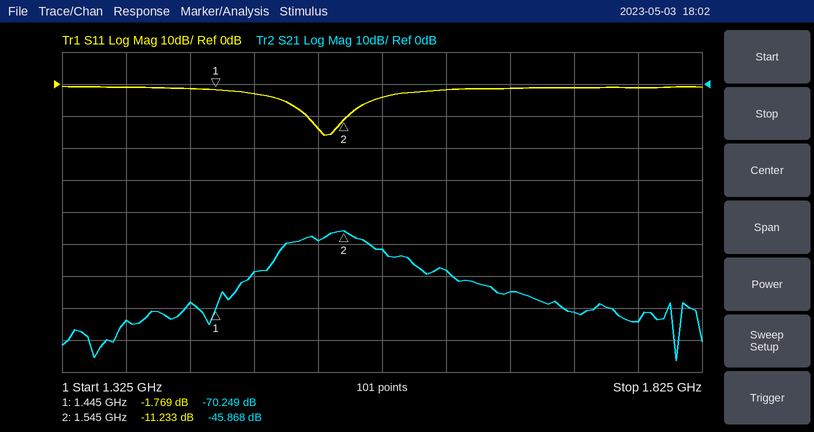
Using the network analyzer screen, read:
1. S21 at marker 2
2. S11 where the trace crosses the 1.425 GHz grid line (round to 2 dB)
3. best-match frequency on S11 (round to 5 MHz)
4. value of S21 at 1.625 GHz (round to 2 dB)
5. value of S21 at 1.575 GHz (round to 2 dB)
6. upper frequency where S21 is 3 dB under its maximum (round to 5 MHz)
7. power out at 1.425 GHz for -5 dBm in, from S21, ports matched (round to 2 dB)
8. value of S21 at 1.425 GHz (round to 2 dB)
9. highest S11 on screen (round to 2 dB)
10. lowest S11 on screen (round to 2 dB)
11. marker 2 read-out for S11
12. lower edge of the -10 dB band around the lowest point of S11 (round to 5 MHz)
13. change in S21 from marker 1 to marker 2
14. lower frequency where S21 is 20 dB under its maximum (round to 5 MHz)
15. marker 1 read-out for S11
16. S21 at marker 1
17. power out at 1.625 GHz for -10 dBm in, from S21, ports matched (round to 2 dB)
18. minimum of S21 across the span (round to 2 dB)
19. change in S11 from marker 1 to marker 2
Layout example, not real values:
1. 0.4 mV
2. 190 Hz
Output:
1. -45.868 dB
2. -2 dB
3. 1.530 GHz
4. -58 dB
5. -52 dB
6. 1.560 GHz
7. -74 dBm
8. -68 dB
9. 0 dB
10. -16 dB
11. -11.233 dB
12. 1.515 GHz
13. 24.381 dB
14. 1.460 GHz
15. -1.769 dB
16. -70.249 dB
17. -68 dBm
18. -86 dB
19. -9.464 dB
